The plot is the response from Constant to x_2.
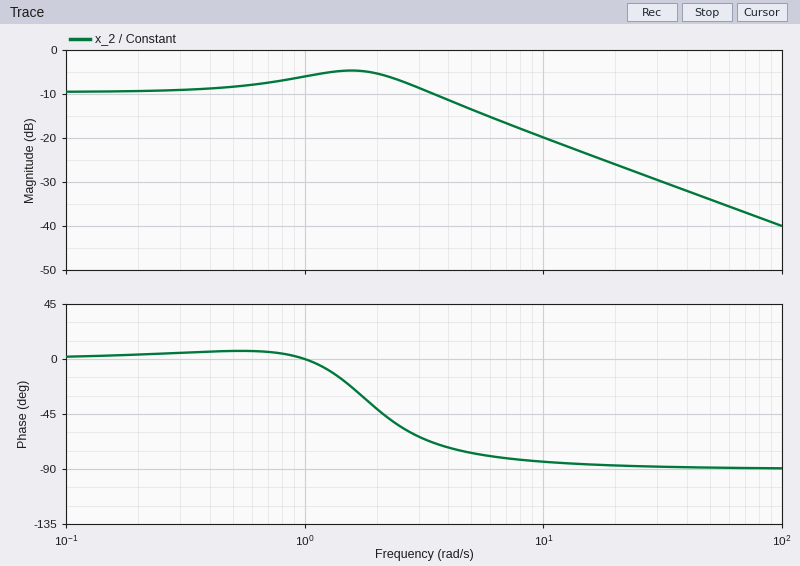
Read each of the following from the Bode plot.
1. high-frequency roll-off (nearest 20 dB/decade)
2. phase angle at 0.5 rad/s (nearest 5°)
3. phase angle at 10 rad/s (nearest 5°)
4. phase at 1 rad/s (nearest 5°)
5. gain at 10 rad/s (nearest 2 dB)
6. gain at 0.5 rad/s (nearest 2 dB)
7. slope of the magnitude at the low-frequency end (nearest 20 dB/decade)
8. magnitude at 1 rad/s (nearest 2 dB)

-20 dB/decade
5°
-85°
0°
-20 dB
-8 dB
0 dB/decade
-6 dB
